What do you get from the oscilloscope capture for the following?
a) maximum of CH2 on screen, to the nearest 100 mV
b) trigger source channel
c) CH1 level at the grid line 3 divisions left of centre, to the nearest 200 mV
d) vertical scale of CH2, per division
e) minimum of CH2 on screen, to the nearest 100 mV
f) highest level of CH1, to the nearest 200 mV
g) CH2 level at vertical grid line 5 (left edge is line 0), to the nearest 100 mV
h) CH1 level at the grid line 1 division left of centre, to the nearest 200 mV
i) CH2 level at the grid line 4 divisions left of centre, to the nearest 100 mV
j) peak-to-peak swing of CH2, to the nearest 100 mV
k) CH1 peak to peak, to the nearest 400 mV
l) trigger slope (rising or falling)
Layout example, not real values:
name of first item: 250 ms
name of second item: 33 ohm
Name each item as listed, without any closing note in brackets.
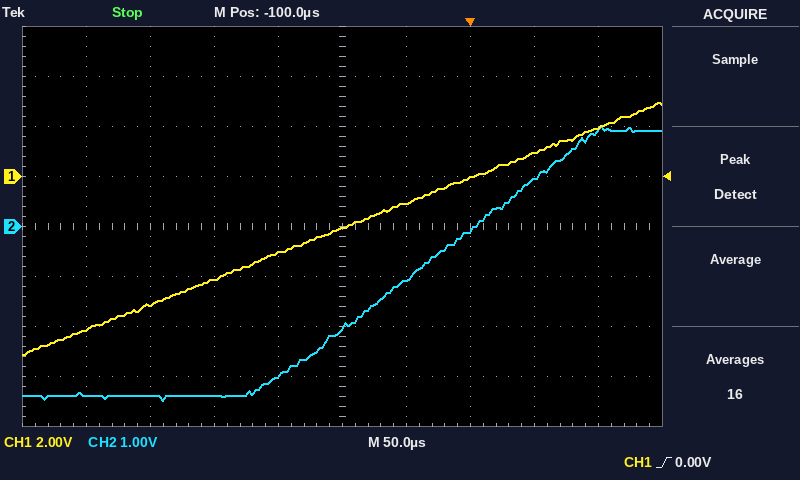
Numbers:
maximum of CH2 on screen, to the nearest 100 mV: 2.0 V
trigger source channel: CH1
CH1 level at the grid line 3 divisions left of centre, to the nearest 200 mV: -5.2 V
vertical scale of CH2, per division: 1 V
minimum of CH2 on screen, to the nearest 100 mV: -3.5 V
highest level of CH1, to the nearest 200 mV: 3.0 V
CH2 level at vertical grid line 5 (left edge is line 0), to the nearest 100 mV: -2.0 V
CH1 level at the grid line 1 division left of centre, to the nearest 200 mV: -3.0 V
CH2 level at the grid line 4 divisions left of centre, to the nearest 100 mV: -3.4 V
peak-to-peak swing of CH2, to the nearest 100 mV: 5.5 V
CH1 peak to peak, to the nearest 400 mV: 10.0 V
trigger slope: rising
